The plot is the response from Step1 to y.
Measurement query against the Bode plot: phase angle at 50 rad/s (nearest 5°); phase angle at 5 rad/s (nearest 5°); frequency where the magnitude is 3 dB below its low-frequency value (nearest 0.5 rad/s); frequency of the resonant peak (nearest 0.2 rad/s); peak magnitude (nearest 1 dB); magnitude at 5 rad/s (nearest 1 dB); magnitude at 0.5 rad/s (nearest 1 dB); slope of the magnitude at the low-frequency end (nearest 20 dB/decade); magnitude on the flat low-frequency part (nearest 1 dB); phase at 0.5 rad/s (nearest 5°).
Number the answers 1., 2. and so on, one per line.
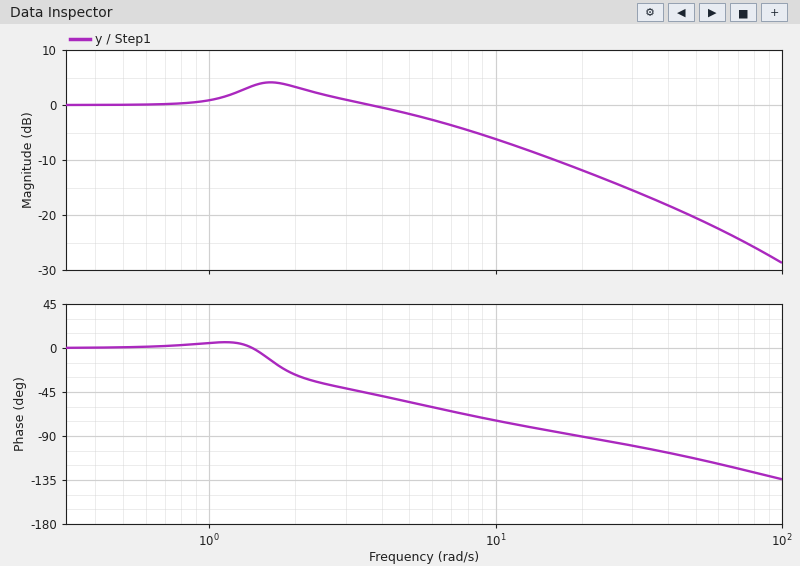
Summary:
1. -115°
2. -55°
3. 6.5 rad/s
4. 1.6 rad/s
5. 4 dB
6. -2 dB
7. 0 dB
8. 0 dB/decade
9. 0 dB
10. 0°
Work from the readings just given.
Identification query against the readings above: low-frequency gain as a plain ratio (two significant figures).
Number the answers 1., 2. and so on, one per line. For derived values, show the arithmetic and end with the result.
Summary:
1. 10^(0 / 20) = 1.0
